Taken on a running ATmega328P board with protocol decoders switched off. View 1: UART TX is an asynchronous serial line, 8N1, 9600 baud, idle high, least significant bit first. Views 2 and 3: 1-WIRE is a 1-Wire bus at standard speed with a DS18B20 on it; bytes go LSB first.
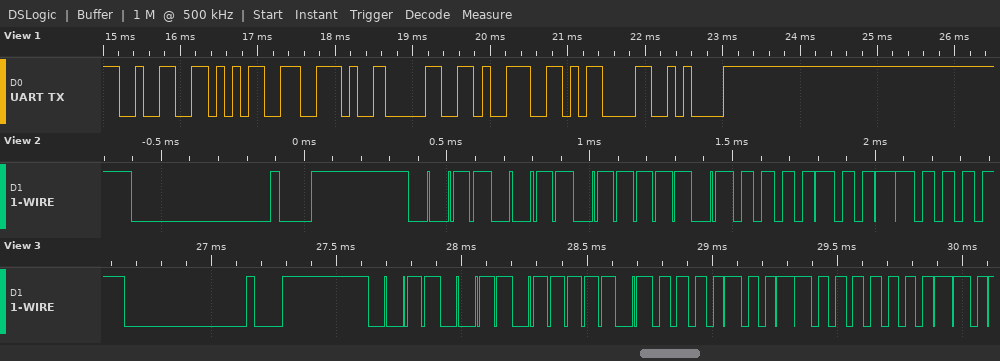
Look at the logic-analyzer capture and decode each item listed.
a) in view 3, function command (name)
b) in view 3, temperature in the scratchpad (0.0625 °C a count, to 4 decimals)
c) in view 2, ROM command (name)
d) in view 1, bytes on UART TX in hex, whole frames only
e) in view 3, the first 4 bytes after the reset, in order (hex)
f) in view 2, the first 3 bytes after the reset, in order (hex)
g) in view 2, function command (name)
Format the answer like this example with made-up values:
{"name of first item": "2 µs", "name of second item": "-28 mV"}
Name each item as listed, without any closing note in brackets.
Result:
{"in view 3, function command": "Read Scratchpad", "in view 3, temperature in the scratchpad": "25.0000 °C", "in view 2, ROM command": "Skip ROM", "in view 1, bytes on UART TX in hex, whole frames only": "32 35 2E 30 39 0D 0A", "in view 3, the first 4 bytes after the reset, in order": "CC BE 90 01", "in view 2, the first 3 bytes after the reset, in order": "CC BE 90", "in view 2, function command": "Read Scratchpad"}
